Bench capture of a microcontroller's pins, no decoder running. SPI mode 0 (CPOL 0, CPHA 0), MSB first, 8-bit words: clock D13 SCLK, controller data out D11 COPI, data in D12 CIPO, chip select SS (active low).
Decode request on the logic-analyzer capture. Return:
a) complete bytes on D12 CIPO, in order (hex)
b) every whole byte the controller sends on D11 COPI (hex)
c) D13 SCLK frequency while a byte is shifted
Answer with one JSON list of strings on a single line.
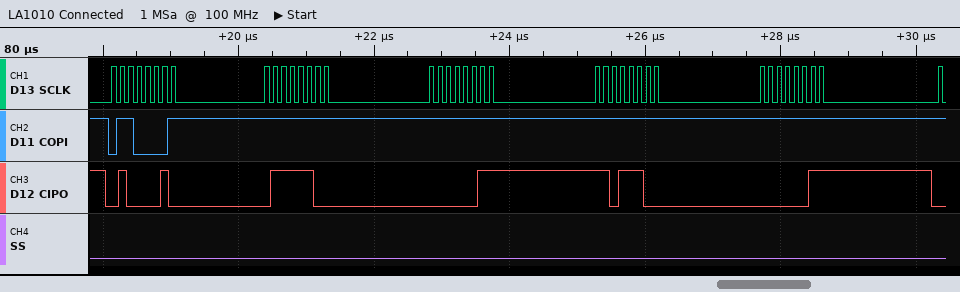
["0x42 0x7C 0x03 0xDC 0x03", "0x61 0xFF 0xFF 0xFF 0xFF", "8 MHz"]
